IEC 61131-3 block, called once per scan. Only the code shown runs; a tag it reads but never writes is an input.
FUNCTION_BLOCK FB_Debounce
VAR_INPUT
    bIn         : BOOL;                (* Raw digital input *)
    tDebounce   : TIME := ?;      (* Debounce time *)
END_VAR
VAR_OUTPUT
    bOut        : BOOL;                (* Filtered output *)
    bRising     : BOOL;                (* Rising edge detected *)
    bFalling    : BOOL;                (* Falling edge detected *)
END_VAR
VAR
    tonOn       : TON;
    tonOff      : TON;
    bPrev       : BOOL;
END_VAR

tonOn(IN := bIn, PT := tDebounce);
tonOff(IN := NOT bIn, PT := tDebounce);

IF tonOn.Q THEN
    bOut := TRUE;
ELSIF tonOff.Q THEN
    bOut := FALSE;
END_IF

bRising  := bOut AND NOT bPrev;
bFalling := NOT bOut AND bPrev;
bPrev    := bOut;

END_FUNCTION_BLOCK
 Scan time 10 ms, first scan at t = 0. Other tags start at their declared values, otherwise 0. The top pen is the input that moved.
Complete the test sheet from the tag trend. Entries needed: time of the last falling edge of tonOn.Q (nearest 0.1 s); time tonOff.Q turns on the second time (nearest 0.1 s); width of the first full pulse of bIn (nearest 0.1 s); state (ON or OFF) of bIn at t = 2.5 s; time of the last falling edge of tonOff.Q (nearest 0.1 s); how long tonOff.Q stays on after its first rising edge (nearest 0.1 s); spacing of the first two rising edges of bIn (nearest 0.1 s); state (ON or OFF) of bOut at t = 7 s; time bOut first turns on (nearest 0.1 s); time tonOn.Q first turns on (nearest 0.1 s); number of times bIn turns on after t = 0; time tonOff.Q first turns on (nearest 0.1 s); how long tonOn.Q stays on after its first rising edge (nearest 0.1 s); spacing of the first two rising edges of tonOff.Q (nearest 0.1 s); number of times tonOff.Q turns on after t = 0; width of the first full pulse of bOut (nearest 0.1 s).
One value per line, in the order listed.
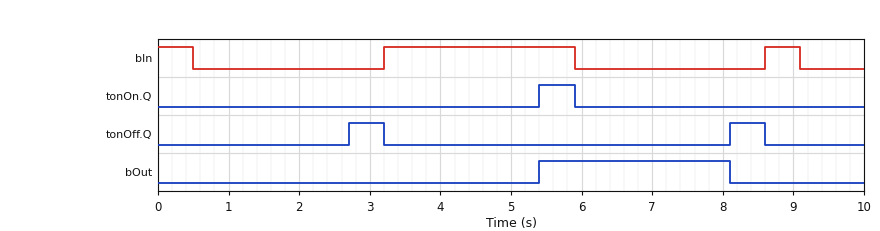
5.9 s
8.1 s
2.7 s
OFF
8.6 s
0.5 s
5.4 s
ON
5.4 s
5.4 s
2
2.7 s
0.5 s
5.4 s
2
2.7 s
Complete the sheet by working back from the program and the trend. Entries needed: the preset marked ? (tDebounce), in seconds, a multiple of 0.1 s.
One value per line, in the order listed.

2.2 s
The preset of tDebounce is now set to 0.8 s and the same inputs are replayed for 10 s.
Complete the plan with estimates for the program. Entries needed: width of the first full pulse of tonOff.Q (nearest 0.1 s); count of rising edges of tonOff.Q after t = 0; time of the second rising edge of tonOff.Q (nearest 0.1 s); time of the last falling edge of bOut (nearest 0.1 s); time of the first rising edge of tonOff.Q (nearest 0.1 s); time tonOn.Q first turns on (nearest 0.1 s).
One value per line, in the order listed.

1.9 s
3
6.7 s
6.7 s
1.3 s
4.0 s
